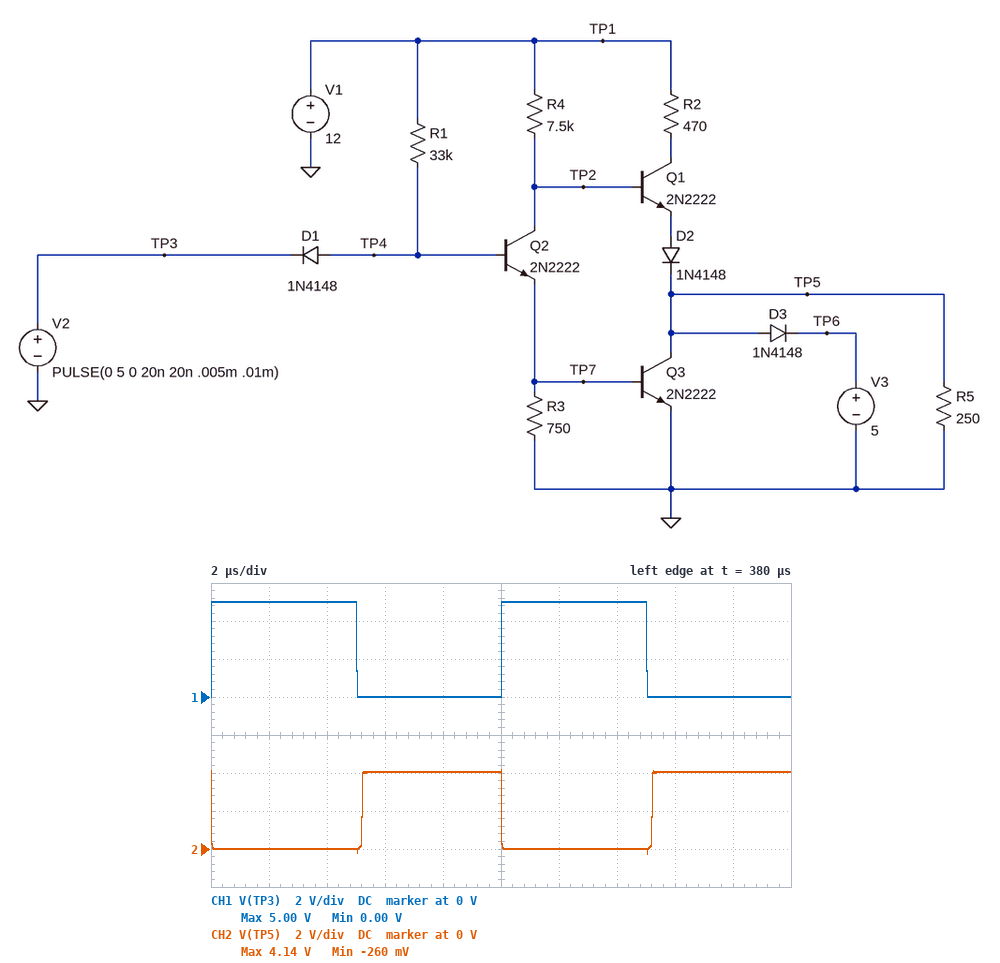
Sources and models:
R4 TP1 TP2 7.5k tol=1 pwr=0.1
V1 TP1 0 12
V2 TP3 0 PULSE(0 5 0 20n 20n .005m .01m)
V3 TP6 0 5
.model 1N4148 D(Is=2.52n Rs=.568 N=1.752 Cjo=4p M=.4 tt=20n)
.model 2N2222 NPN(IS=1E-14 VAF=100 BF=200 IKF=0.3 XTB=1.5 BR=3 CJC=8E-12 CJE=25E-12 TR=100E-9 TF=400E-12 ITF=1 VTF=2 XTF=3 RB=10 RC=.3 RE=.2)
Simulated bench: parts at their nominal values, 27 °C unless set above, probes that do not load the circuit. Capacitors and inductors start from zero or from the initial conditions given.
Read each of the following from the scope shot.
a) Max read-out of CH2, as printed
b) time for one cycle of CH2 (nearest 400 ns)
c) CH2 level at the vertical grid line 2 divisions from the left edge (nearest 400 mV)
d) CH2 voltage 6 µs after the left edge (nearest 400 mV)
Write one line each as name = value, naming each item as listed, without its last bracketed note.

Max read-out of CH2, as printed = 4.14 V
time for one cycle of CH2 = 10.0 µs
CH2 level at the vertical grid line 2 divisions from the left edge = 0 V
CH2 voltage 6 µs after the left edge = 4.0 V
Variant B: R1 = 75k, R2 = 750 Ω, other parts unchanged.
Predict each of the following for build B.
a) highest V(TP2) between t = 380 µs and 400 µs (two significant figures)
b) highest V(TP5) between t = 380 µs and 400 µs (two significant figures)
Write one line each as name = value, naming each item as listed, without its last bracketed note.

highest V(TP2) between t = 380 µs and 400 µs = 4.5 V
highest V(TP5) between t = 380 µs and 400 µs = 3.1 V
